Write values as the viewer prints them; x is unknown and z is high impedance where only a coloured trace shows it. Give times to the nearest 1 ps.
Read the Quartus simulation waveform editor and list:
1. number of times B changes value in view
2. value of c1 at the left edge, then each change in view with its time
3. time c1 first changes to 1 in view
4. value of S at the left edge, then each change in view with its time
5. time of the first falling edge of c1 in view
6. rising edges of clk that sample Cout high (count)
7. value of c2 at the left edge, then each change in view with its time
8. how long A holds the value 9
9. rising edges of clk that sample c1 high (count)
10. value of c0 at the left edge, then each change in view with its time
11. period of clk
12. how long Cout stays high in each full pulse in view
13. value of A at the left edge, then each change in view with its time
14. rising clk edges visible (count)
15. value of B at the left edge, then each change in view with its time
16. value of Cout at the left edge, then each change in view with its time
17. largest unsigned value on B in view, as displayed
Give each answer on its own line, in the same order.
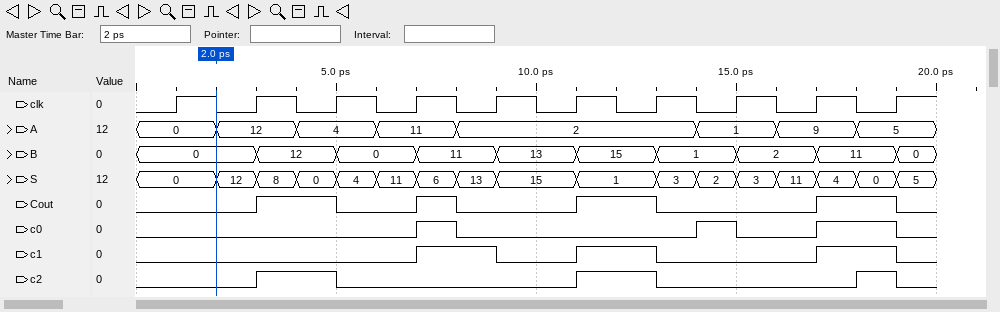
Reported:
9
0, 1 at 7 ps, 0 at 9 ps, 1 at 11 ps, 0 at 13 ps, 1 at 17 ps, 0 at 19 ps
7 ps
0, 12 at 2 ps, 8 at 3 ps, 0 at 4 ps, 4 at 5 ps, 11 at 6 ps, 6 at 7 ps, 13 at 8 ps, 15 at 9 ps, 1 at 11 ps, 3 at 13 ps, 2 at 14 ps, 3 at 15 ps, 11 at 16 ps, 4 at 17 ps, 0 at 18 ps, 5 at 19 ps
9 ps
3
0, 1 at 3 ps, 0 at 5 ps, 1 at 11 ps, 0 at 13 ps, 1 at 18 ps, 0 at 19 ps
2 ps
3
0, 1 at 7 ps, 0 at 8 ps, 1 at 14 ps, 0 at 15 ps, 1 at 17 ps, 0 at 19 ps
2 ps
2 ps, 1 ps, 2 ps, 2 ps
0, 12 at 2 ps, 4 at 4 ps, 11 at 6 ps, 2 at 8 ps, 1 at 14 ps, 9 at 16 ps, 5 at 18 ps
10
0, 12 at 3 ps, 0 at 5 ps, 11 at 7 ps, 13 at 9 ps, 15 at 11 ps, 1 at 13 ps, 2 at 15 ps, 11 at 17 ps, 0 at 19 ps
0, 1 at 3 ps, 0 at 5 ps, 1 at 7 ps, 0 at 8 ps, 1 at 11 ps, 0 at 13 ps, 1 at 17 ps, 0 at 19 ps
15
